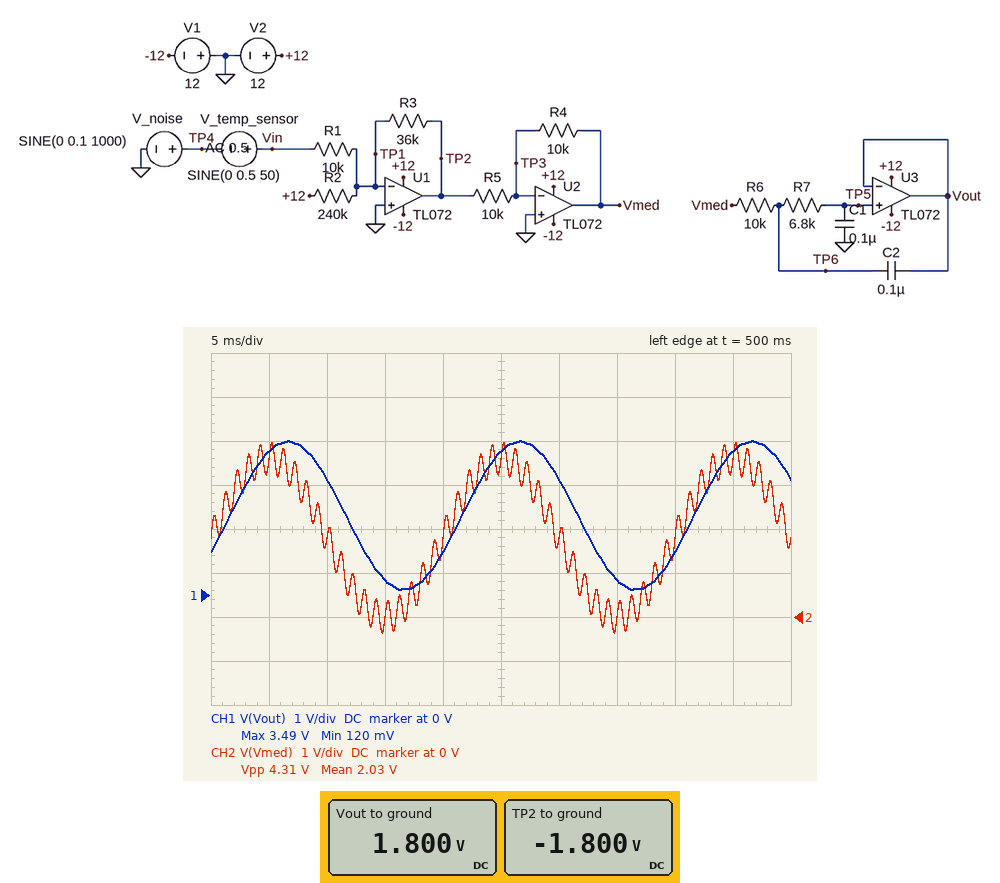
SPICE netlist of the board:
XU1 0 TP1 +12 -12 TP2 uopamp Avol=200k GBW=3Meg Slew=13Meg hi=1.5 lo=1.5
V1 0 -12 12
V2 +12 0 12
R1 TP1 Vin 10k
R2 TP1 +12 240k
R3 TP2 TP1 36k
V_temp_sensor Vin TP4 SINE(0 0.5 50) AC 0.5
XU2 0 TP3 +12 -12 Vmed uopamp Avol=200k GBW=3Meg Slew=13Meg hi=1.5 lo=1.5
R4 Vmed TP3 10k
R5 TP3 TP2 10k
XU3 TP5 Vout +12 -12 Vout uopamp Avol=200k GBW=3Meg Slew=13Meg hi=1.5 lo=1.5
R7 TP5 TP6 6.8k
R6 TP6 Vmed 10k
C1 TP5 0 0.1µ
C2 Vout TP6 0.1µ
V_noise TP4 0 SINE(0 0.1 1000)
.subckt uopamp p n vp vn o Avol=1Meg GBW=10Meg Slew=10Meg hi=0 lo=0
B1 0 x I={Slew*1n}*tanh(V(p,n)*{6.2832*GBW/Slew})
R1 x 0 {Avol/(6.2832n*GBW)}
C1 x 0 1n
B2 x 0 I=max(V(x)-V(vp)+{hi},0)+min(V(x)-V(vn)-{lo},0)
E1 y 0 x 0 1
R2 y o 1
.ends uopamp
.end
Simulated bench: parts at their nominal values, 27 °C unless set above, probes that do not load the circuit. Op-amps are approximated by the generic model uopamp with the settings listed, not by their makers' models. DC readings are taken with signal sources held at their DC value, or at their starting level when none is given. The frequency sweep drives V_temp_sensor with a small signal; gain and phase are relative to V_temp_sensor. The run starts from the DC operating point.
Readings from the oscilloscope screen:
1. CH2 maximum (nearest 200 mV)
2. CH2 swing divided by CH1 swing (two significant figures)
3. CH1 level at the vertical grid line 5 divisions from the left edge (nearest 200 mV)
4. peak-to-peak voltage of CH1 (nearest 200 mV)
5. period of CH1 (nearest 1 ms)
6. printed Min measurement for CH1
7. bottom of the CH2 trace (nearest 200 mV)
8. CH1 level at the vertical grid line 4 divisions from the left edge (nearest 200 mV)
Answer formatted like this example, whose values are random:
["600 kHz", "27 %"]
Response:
["4.0 V", "1.3", "3.2 V", "3.4 V", "20 ms", "120 mV", "-400 mV", "1.0 V"]
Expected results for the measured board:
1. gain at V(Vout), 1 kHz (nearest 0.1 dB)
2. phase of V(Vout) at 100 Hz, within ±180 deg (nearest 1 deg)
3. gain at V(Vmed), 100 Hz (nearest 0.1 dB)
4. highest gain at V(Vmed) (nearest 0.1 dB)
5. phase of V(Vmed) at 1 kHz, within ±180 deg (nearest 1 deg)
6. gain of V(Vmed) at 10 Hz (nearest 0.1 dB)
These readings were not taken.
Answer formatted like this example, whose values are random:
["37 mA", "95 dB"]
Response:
["-17.8 dB", "-55 deg", "11.1 dB", "11.1 dB", "0 deg", "11.1 dB"]
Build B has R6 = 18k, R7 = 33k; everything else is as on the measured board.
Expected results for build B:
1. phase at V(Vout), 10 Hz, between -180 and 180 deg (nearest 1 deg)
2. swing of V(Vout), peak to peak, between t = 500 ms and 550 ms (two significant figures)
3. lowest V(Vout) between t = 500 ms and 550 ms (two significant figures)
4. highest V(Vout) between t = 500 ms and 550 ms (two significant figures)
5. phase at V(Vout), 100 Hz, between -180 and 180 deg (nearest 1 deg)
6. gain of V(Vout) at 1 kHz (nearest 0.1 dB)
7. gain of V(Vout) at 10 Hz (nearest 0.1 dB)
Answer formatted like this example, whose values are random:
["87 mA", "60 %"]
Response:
["-18 deg", "2.2 V", "710 mV", "2.9 V", "-113 deg", "-36.3 dB", "10.9 dB"]
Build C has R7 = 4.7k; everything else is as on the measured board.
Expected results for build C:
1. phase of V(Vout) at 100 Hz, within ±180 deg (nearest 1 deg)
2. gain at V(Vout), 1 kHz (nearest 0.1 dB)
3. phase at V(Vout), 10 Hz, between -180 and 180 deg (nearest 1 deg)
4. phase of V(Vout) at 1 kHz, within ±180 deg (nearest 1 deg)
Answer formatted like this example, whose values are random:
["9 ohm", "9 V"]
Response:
["-49 deg", "-14.8 dB", "-5 deg", "-152 deg"]
